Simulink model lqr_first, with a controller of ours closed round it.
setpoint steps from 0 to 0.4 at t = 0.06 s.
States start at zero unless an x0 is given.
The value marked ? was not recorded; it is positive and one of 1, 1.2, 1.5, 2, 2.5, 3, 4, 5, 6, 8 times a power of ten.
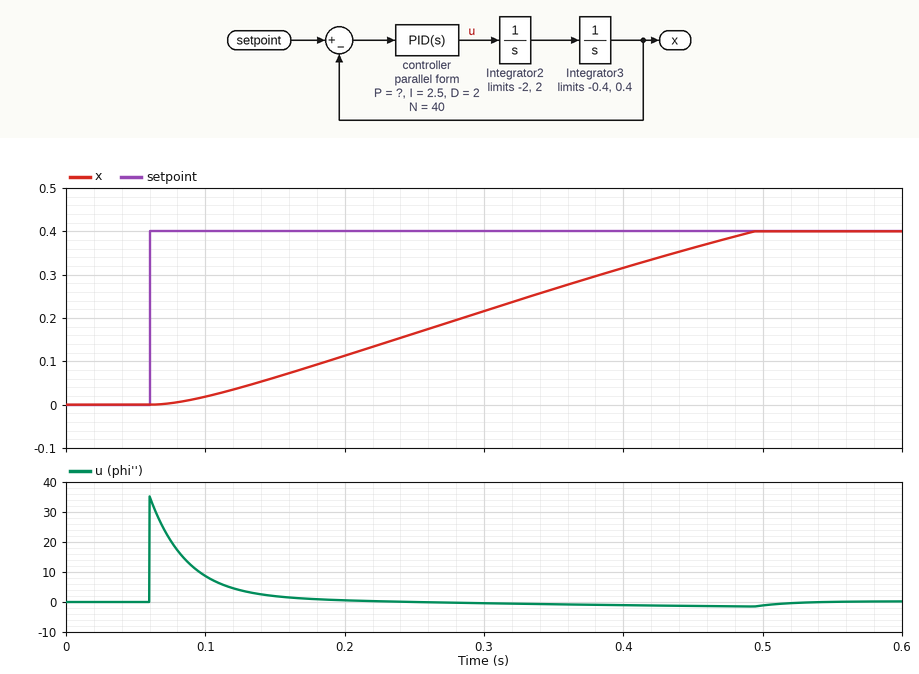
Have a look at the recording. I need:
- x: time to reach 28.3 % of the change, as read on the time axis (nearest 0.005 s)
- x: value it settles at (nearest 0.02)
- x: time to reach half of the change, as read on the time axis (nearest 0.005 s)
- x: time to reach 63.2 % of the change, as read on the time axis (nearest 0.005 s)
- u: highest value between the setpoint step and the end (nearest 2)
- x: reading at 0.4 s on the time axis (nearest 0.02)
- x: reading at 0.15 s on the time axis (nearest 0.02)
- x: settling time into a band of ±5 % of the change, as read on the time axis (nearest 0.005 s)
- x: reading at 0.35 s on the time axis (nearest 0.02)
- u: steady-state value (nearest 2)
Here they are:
0.200 s
0.40
0.285 s
0.335 s
34
0.32
0.06
0.470 s
0.26
0
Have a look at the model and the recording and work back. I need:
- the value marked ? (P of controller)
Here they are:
8
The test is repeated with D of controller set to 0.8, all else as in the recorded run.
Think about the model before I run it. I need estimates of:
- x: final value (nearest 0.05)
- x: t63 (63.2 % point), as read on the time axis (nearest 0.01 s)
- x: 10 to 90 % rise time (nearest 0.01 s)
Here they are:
0.40
0.41 s
0.35 s
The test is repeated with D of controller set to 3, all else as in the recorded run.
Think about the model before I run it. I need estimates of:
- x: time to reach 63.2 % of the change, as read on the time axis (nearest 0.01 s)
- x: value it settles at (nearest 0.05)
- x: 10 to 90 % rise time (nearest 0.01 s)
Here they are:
0.29 s
0.40
0.29 s
